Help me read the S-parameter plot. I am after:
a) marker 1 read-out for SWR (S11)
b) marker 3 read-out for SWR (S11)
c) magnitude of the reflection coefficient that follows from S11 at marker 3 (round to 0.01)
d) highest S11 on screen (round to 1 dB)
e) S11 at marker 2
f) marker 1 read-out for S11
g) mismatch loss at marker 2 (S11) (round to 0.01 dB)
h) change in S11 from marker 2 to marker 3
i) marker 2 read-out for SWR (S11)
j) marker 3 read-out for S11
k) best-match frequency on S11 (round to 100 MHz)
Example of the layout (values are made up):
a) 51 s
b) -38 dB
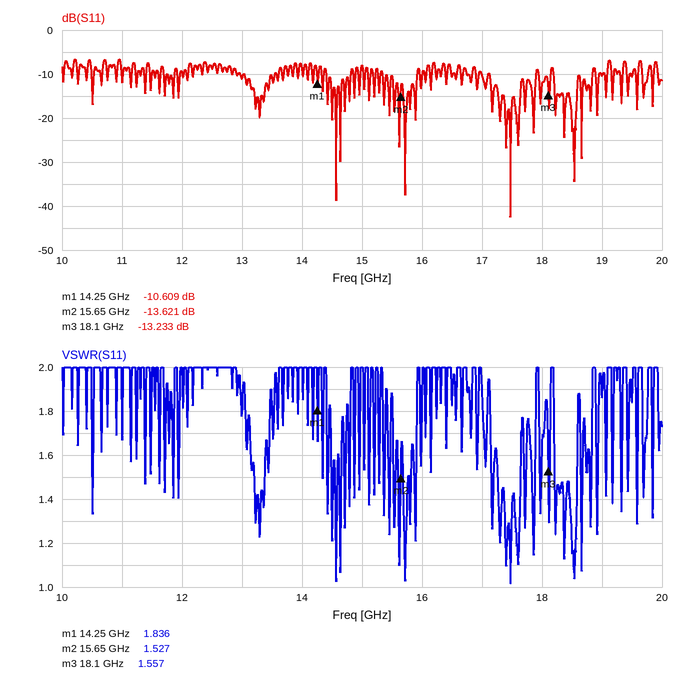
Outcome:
a) 1.836
b) 1.557
c) 0.22
d) -7 dB
e) -13.621 dB
f) -10.609 dB
g) 0.19 dB
h) 0.388 dB
i) 1.527
j) -13.233 dB
k) 17.5 GHz
